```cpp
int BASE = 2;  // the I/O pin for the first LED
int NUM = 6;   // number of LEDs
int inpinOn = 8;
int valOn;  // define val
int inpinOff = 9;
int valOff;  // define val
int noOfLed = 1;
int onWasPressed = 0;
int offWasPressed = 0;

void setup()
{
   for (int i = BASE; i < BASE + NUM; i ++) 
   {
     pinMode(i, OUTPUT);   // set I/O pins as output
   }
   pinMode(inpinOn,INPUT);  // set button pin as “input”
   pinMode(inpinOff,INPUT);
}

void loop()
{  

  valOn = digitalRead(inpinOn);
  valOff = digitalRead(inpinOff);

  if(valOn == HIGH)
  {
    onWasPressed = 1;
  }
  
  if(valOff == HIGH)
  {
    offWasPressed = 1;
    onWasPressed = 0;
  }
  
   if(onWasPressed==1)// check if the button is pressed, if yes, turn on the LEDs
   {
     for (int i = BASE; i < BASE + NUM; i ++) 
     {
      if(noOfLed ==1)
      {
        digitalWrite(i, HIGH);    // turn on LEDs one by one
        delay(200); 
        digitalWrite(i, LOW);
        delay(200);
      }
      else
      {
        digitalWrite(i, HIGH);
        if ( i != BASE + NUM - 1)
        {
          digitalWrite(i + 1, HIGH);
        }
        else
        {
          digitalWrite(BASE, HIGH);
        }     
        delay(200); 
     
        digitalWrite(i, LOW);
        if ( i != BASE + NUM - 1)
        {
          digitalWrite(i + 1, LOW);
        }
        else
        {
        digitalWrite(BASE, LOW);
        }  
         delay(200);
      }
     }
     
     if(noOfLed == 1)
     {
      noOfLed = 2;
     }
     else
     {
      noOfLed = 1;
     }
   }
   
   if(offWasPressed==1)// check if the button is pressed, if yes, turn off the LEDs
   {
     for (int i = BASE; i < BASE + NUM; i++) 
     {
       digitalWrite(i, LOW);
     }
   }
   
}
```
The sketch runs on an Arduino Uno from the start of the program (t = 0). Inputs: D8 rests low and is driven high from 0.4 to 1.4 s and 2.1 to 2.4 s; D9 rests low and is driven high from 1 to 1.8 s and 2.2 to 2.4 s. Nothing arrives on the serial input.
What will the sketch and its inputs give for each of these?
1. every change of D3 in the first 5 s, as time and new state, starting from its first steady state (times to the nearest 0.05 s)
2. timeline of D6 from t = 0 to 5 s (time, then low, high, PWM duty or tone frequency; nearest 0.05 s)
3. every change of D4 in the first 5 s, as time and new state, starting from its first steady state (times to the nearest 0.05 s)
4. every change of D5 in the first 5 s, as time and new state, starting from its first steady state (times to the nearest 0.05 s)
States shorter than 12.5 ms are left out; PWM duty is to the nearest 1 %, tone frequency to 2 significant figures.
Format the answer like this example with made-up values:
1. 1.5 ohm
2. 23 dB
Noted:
1. 0 s low; 0.8 s high; 1 s low; 2.8 s high; 3 s low; 3.2 s high; 3.4 s low
2. 0 s low; 2 s high; 2.2 s low; 4 s high; 4.2 s low; 4.4 s high; 4.6 s low
3. 0 s low; 1.2 s high; 1.4 s low; 3.2 s high; 3.4 s low; 3.6 s high; 3.8 s low
4. 0 s low; 1.6 s high; 1.8 s low; 3.6 s high; 3.8 s low; 4 s high; 4.2 s low
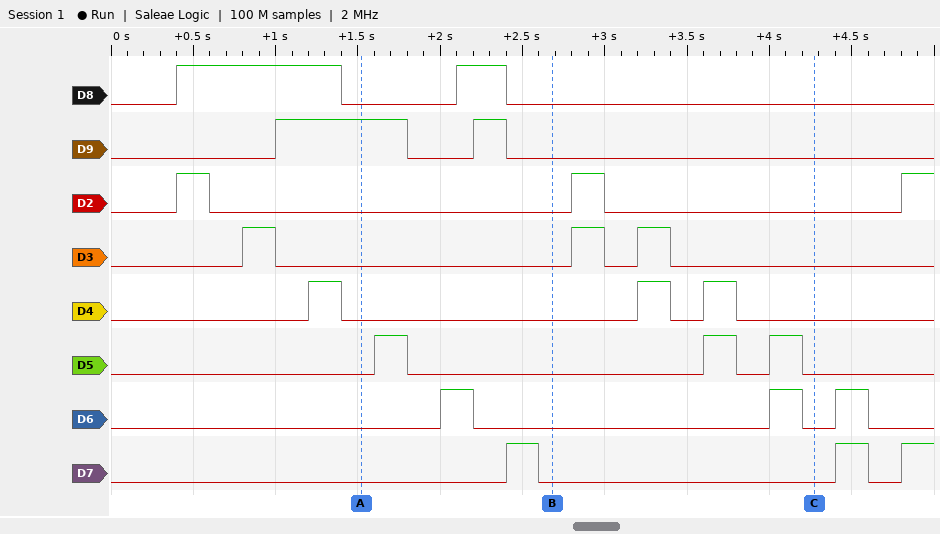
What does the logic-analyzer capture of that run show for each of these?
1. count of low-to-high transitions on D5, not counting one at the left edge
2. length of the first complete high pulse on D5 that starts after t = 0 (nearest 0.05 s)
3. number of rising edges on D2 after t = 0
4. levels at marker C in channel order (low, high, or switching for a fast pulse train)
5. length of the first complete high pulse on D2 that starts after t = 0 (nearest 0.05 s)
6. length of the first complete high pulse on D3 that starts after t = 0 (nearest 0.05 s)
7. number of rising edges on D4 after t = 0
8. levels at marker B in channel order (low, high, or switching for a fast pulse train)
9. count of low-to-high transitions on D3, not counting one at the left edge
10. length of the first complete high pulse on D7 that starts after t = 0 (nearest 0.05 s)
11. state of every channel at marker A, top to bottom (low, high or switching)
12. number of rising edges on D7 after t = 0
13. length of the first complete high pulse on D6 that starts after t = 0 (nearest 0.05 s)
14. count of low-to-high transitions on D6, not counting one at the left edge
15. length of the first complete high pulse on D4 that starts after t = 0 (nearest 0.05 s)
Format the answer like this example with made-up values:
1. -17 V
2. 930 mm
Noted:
1. 3
2. 0.20 s
3. 3
4. D8 low, D9 low, D2 low, D3 low, D4 low, D5 low, D6 low, D7 low
5. 0.20 s
6. 0.20 s
7. 3
8. D8 low, D9 low, D2 low, D3 low, D4 low, D5 low, D6 low, D7 low
9. 3
10. 0.20 s
11. D8 low, D9 high, D2 low, D3 low, D4 low, D5 low, D6 low, D7 low
12. 3
13. 0.20 s
14. 3
15. 0.20 s
